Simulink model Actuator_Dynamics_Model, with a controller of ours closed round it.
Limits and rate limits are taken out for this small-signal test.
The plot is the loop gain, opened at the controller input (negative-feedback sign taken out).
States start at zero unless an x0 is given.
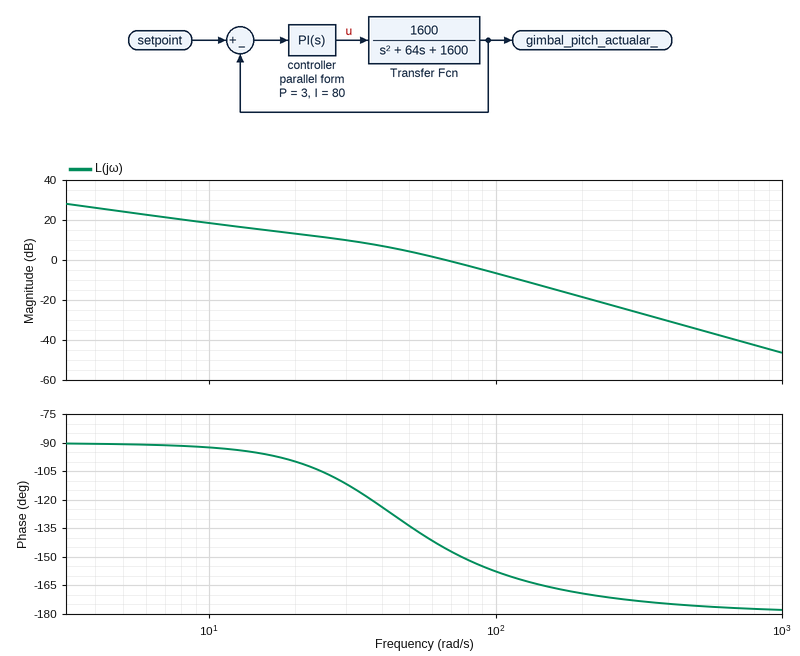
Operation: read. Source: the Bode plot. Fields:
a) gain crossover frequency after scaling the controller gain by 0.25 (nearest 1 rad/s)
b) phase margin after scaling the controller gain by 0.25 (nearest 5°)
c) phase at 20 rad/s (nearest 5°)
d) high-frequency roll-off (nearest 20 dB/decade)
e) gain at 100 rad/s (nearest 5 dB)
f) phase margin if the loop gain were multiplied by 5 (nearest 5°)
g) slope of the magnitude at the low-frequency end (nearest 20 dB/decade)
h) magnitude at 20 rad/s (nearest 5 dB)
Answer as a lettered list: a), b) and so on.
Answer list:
a) 23 rad/s
b) 75°
c) -100°
d) -40 dB/decade
e) -5 dB
f) 15°
g) -20 dB/decade
h) 15 dB
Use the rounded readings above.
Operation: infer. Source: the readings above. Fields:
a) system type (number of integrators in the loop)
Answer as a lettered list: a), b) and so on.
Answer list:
a) 1
